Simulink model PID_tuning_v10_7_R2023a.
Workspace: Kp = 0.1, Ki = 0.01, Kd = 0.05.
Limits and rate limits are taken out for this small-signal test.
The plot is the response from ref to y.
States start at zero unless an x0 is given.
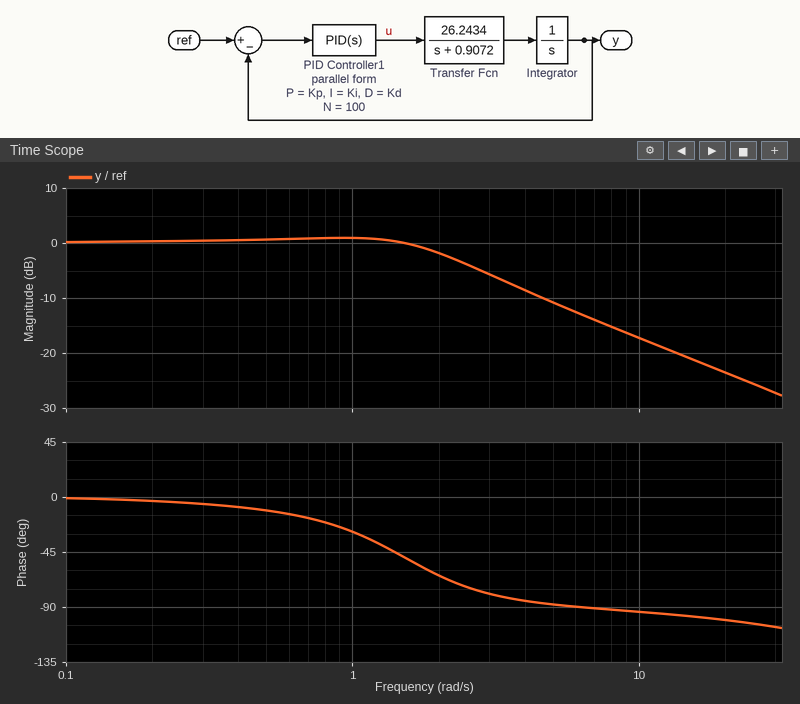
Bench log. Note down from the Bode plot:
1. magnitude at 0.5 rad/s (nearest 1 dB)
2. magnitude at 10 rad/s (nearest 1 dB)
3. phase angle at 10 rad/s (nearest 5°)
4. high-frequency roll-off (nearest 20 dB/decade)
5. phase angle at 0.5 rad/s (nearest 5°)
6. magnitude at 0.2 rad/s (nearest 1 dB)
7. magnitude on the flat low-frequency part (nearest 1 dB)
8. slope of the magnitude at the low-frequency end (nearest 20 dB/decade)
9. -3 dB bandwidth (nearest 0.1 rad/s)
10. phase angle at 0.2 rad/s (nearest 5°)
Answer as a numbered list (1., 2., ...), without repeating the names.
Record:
1. 1 dB
2. -17 dB
3. -95°
4. -20 dB/decade
5. -10°
6. 0 dB
7. 0 dB
8. 0 dB/decade
9. 2.2 rad/s
10. -5°
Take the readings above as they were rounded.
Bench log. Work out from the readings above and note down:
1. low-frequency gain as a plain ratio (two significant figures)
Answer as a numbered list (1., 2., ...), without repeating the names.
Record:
1. 1.0
